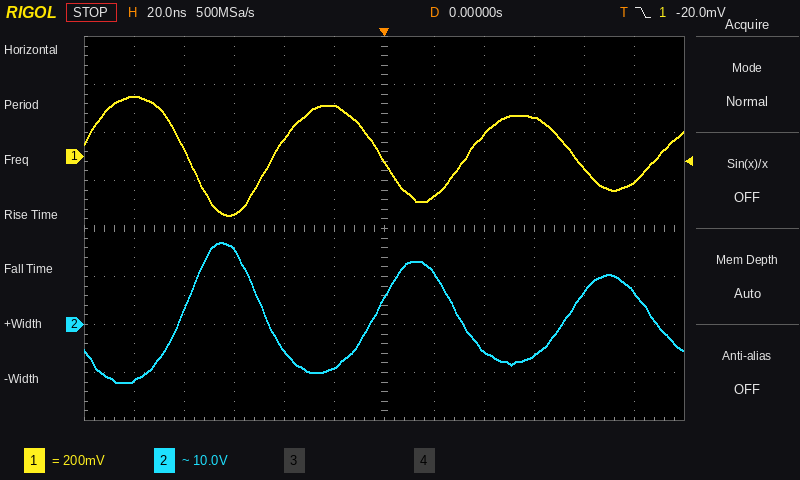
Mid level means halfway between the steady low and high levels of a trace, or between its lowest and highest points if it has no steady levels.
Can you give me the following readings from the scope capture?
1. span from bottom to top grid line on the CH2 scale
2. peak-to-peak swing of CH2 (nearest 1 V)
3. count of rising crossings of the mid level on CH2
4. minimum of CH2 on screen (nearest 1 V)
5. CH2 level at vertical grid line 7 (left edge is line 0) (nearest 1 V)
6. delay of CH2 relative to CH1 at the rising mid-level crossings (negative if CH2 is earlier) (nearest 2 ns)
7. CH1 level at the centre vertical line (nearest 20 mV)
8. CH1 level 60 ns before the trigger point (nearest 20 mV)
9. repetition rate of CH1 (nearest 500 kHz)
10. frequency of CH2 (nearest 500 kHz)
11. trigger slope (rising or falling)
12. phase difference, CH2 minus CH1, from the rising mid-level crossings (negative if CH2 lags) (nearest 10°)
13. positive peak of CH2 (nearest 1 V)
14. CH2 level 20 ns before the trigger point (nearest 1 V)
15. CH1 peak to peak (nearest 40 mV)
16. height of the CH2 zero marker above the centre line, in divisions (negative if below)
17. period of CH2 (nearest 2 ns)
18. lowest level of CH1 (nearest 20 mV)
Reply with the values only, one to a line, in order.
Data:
80 V
29 V
3
-12 V
11 V
-36 ns
-20 mV
-240 mV
13.0 MHz
13.0 MHz
falling
+170°
17 V
-9 V
480 mV
-2.0 div
78 ns
-240 mV
